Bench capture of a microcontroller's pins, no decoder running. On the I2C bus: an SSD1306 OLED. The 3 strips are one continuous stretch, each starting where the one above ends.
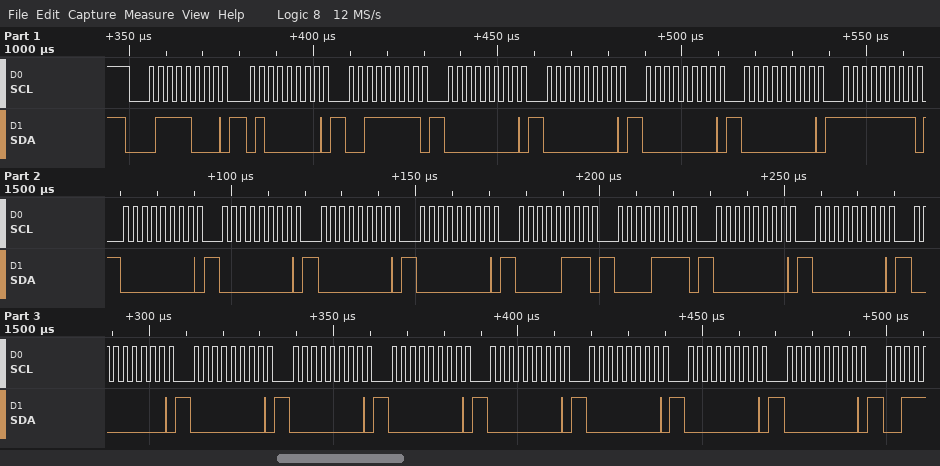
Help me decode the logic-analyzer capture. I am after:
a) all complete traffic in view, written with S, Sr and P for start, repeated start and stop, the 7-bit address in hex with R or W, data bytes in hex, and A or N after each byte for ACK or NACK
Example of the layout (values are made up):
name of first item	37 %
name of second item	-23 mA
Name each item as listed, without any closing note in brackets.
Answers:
all complete traffic in view, written with S, Sr and P for start, repeated start and stop, the 7-bit address in hex with R or W, data bytes in hex, and A or N after each byte for ACK or NACK	S 3CW A 40 A 3F A 00 A 00 A 00 A 00 A FF A 00 A 00 A 00 A 00 A 07 A 0F A 00 A 00 A 00 A 00 A 00 A 00 A 00 A 00 A 00 A 00 A
